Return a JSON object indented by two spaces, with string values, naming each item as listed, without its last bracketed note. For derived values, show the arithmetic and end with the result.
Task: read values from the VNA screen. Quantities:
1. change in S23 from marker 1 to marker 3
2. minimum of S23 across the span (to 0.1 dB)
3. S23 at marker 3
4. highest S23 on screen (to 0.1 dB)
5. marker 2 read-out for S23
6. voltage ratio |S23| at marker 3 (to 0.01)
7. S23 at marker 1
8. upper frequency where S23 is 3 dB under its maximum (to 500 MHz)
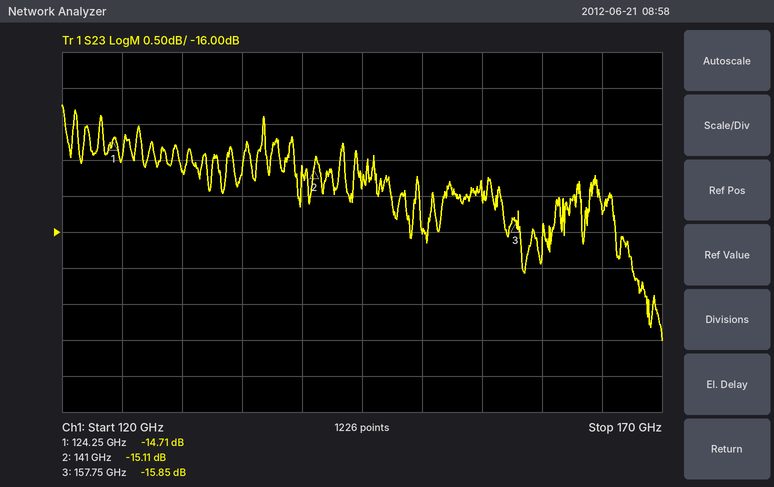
{
  "change in S23 from marker 1 to marker 3": "-15.85 − (-14.71) = -1.14 dB",
  "minimum of S23 across the span": "-17.5 dB",
  "S23 at marker 3": "-15.85 dB",
  "highest S23 on screen": "-14.2 dB",
  "marker 2 read-out for S23": "-15.11 dB",
  "voltage ratio |S23| at marker 3": "10^(-15.85/20) ≈ 0.16",
  "S23 at marker 1": "-14.71 dB",
  "upper frequency where S23 is 3 dB under its maximum": "169.0 GHz"
}
